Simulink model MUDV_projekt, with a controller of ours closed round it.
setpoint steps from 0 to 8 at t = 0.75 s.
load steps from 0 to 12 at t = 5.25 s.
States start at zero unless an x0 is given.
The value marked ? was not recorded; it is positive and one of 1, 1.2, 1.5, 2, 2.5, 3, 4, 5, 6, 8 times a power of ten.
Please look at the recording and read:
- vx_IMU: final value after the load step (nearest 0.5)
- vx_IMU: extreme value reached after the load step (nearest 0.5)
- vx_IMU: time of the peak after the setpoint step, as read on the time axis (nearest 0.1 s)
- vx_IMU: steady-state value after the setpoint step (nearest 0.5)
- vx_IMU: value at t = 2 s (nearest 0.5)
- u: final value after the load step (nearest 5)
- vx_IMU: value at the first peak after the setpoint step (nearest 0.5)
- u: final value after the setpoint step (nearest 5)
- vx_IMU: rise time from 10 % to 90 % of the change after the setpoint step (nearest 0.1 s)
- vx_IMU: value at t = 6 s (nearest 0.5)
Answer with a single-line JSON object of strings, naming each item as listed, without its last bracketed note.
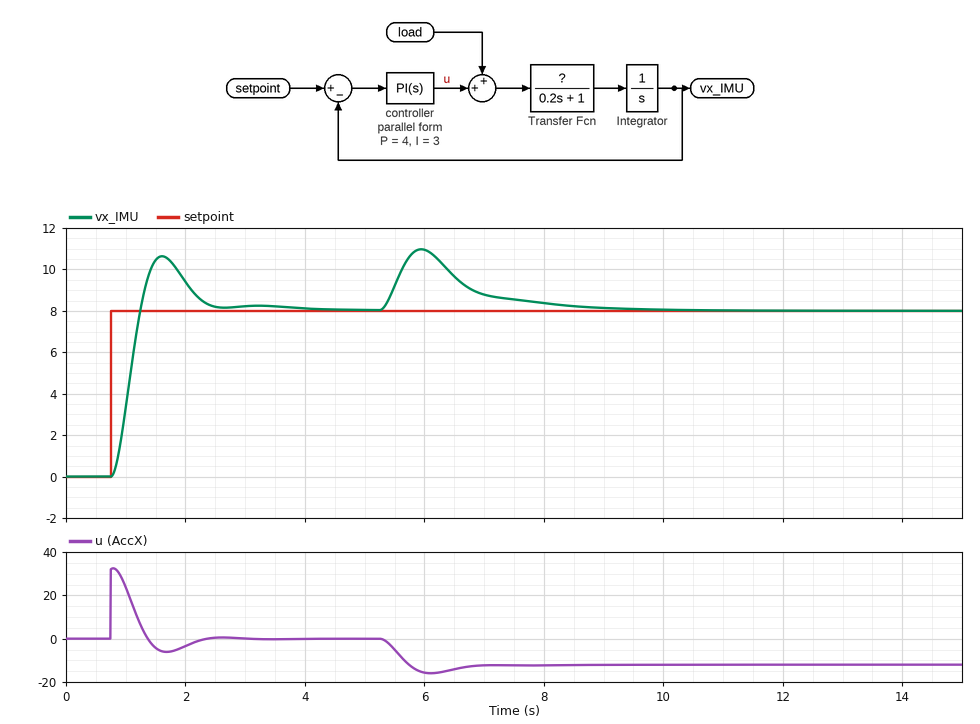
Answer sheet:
{"vx_IMU: final value after the load step": "8.0", "vx_IMU: extreme value reached after the load step": "11.0", "vx_IMU: time of the peak after the setpoint step, as read on the time axis": "1.6 s", "vx_IMU: steady-state value after the setpoint step": "8.0", "vx_IMU: value at t = 2 s": "9.5", "u: final value after the load step": "-10", "vx_IMU: value at the first peak after the setpoint step": "10.5", "u: final value after the setpoint step": "0", "vx_IMU: rise time from 10 % to 90 % of the change after the setpoint step": "0.3 s", "vx_IMU: value at t = 6 s": "11.0"}
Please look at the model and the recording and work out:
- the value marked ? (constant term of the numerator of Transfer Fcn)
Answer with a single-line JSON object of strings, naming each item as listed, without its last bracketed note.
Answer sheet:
{"the value marked ?": "1"}
